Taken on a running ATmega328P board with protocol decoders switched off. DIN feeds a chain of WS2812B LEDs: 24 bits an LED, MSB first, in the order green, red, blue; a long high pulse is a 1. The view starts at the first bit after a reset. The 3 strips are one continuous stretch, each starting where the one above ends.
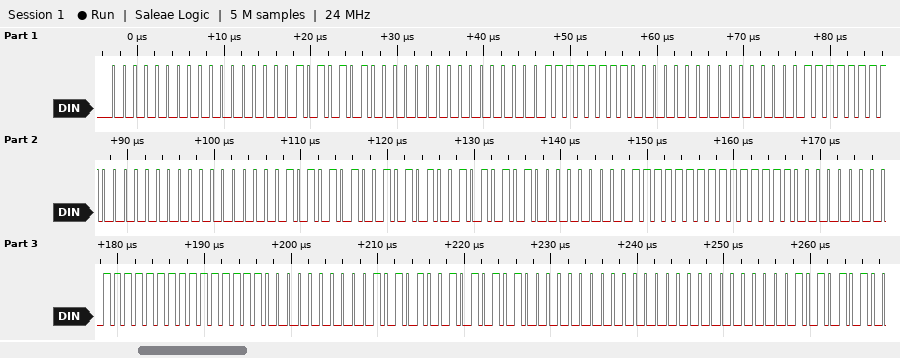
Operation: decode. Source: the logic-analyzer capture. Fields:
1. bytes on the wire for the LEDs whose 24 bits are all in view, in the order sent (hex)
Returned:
00 00 55 00 00 FF 00 00 FF 00 00 55 2A 55 00 7F FF 00 7F FF 00 2A 55 00 00 00 55
